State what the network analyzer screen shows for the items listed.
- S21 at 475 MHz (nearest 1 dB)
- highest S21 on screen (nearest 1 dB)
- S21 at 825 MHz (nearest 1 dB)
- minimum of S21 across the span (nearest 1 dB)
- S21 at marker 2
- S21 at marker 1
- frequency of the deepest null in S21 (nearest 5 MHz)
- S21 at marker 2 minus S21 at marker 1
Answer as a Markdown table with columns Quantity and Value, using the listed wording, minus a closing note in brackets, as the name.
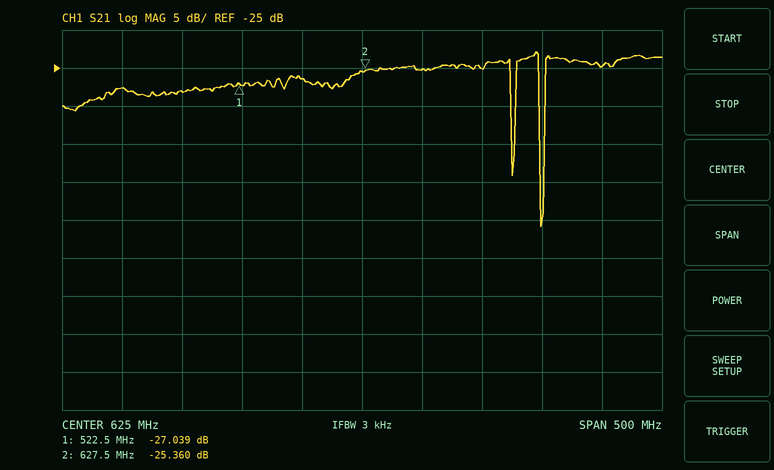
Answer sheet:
| Quantity | Value |
|---|---|
| S21 at 475 MHz | -28 dB |
| highest S21 on screen | -23 dB |
| S21 at 825 MHz | -25 dB |
| minimum of S21 across the span | -46 dB |
| S21 at marker 2 | -25.360 dB |
| S21 at marker 1 | -27.039 dB |
| frequency of the deepest null in S21 | 775 MHz |
| S21 at marker 2 minus S21 at marker 1 | 1.679 dB |
